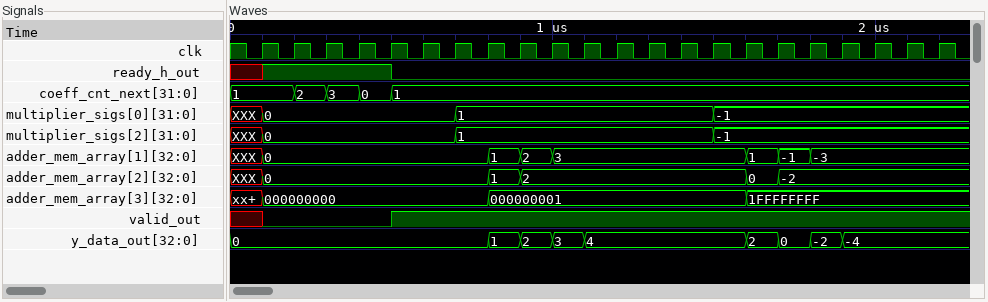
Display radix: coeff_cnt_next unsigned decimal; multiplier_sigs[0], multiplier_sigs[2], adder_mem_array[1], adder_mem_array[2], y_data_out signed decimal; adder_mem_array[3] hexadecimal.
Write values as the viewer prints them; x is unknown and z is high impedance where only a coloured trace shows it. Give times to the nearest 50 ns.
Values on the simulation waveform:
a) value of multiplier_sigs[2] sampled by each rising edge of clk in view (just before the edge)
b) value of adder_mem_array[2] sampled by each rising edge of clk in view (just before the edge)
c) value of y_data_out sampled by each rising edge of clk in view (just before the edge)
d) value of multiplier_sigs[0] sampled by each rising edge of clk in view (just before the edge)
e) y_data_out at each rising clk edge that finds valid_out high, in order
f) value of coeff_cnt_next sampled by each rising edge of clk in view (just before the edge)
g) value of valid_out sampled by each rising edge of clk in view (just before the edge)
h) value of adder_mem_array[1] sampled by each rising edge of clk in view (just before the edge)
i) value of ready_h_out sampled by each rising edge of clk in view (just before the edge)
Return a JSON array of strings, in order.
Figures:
["XXX, 0, 0, 0, 0, 0, 0, 1, 1, 1, 1, 1, 1, 1, 1, -1, -1, -1, -1, -1, -1, -1", "XXX, 0, 0, 0, 0, 0, 0, 0, 1, 2, 2, 2, 2, 2, 2, 2, 0, -2, -2, -2, -2, -2", "0, 0, 0, 0, 0, 0, 0, 0, 1, 2, 3, 4, 4, 4, 4, 4, 2, 0, -2, -4, -4, -4", "XXX, 0, 0, 0, 0, 0, 0, 1, 1, 1, 1, 1, 1, 1, 1, -1, -1, -1, -1, -1, -1, -1", "0, 0, 0, 1, 2, 3, 4, 4, 4, 4, 4, 2, 0, -2, -4, -4, -4", "1, 1, 2, 3, 0, 1, 1, 1, 1, 1, 1, 1, 1, 1, 1, 1, 1, 1, 1, 1, 1, 1", "x 0 0 0 0 1 1 1 1 1 1 1 1 1 1 1 1 1 1 1 1 1", "XXX, 0, 0, 0, 0, 0, 0, 0, 1, 2, 3, 3, 3, 3, 3, 3, 1, -1, -3, -3, -3, -3", "x 1 1 1 1 0 0 0 0 0 0 0 0 0 0 0 0 0 0 0 0 0"]
